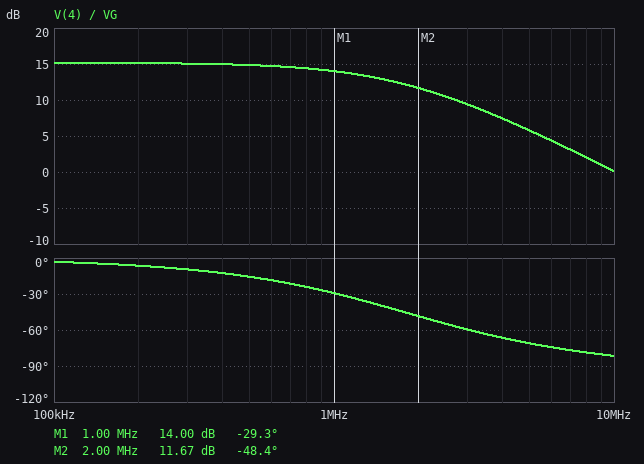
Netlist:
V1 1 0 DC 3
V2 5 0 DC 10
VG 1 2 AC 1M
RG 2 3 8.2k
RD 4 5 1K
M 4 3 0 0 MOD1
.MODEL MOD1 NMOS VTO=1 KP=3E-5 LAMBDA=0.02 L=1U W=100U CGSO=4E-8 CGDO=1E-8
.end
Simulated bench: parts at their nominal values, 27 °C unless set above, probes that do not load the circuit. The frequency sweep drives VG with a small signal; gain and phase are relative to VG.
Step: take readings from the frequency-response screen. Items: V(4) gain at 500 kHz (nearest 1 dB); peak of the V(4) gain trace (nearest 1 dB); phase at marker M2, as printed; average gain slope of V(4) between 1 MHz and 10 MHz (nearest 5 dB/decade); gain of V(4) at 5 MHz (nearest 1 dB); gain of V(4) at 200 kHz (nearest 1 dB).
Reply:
15 dB
15 dB
-48.4 deg
-15 dB/decade
6 dB
15 dB
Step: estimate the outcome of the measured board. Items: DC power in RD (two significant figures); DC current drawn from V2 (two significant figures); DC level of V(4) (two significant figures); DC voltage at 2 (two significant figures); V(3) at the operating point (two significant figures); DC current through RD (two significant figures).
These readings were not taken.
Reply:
41 mW
6.4 mA
3.6 V
3.0 V
3.0 V
6.4 mA
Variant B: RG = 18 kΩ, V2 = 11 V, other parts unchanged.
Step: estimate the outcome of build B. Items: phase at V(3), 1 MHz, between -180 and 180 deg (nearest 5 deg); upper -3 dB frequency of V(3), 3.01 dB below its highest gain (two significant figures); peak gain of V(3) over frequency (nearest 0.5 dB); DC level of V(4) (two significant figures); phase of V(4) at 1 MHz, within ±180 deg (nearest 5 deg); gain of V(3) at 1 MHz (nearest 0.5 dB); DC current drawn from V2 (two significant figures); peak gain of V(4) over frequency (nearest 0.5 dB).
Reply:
130 deg
810 kHz
0 dB
4.5 V
-50 deg
-4.0 dB
6.5 mA
15.5 dB
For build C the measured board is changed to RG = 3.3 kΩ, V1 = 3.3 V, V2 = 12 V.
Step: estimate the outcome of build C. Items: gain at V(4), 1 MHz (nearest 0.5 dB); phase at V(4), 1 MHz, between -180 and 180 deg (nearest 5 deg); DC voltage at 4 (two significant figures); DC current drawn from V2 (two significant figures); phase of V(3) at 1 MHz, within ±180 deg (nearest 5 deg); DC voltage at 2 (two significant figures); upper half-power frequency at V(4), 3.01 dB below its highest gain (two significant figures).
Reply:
16.0 dB
-15 deg
3.5 V
8.5 mA
165 deg
3.3 V
4.2 MHz
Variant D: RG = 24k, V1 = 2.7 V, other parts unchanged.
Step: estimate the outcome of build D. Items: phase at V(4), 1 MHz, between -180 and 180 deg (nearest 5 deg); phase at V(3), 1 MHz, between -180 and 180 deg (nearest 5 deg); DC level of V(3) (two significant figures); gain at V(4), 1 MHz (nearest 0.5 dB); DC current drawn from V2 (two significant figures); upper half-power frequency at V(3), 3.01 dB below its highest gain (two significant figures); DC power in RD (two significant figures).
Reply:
-55 deg
125 deg
2.7 V
9.0 dB
4.8 mA
650 kHz
23 mW
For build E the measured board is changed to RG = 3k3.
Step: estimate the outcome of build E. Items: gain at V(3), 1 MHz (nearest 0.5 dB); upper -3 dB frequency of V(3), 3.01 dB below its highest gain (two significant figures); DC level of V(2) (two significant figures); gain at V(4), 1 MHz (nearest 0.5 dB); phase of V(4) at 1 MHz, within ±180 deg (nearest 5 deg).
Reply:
0 dB
4.4 MHz
3.0 V
15.0 dB
-15 deg
